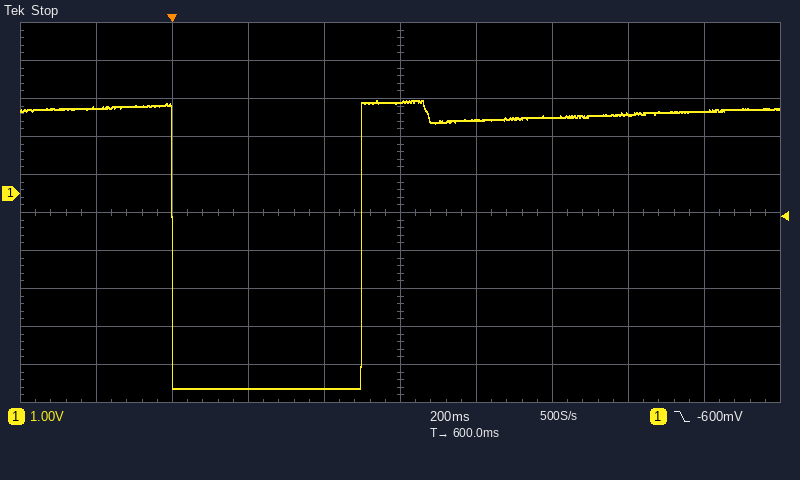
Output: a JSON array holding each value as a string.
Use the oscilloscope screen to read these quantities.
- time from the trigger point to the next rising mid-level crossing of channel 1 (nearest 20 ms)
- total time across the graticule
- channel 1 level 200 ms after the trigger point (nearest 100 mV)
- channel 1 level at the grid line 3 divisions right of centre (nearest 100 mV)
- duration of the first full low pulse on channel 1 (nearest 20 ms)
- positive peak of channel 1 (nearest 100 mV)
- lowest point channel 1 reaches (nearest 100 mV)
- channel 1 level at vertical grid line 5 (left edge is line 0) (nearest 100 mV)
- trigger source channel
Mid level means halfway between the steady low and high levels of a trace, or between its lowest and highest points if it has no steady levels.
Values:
["500 ms", "2 s", "-5.1 V", "2.1 V", "500 ms", "2.4 V", "-5.1 V", "2.4 V", "channel 1"]
